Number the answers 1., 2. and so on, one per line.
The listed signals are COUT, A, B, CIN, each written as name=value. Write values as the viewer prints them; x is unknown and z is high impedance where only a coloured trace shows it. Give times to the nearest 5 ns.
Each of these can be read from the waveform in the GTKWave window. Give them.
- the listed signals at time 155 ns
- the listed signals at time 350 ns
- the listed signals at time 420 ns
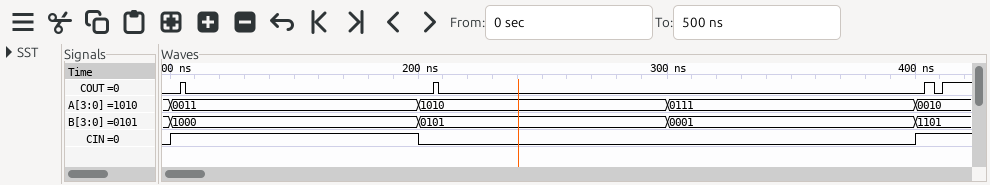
1. COUT=0, A=0011, B=1000, CIN=1
2. COUT=0, A=0111, B=0001, CIN=0
3. COUT=1, A=0010, B=1101, CIN=1
